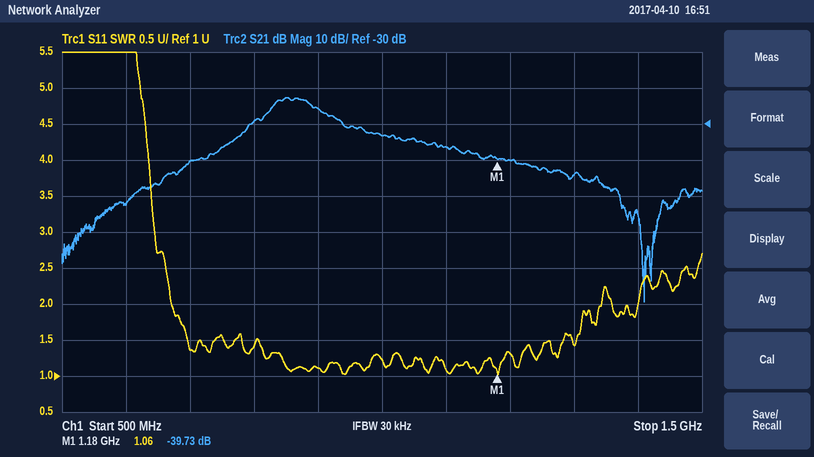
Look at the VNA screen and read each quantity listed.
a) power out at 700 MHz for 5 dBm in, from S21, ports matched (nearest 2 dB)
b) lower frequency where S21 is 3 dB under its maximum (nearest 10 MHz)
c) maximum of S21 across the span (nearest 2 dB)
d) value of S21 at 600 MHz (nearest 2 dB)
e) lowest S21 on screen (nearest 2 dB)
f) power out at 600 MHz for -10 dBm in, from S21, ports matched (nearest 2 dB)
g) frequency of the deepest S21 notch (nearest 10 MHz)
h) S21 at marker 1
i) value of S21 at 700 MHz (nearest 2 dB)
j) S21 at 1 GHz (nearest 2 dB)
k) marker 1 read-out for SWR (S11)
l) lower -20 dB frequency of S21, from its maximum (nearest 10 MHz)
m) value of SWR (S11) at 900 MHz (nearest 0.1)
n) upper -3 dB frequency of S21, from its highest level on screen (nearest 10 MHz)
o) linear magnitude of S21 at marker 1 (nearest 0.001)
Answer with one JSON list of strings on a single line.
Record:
["-36 dBm", "830 MHz", "-22 dB", "-52 dB", "-80 dB", "-62 dBm", "1.41 GHz", "-39.73 dB", "-40 dB", "-34 dB", "1.06", "690 MHz", "1.1", "900 MHz", "0.010"]
